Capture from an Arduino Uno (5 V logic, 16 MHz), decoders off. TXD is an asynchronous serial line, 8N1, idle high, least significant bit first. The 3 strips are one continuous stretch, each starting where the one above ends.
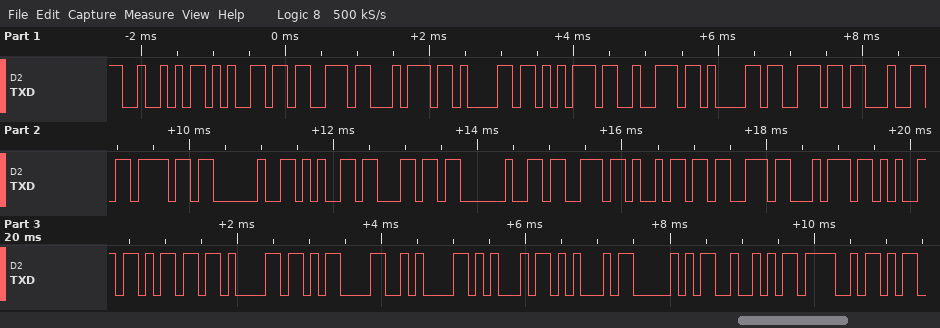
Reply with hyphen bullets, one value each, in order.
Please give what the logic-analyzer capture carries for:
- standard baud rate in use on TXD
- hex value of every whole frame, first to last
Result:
- 9600 baud
- 0x52 0x65 0x73 0x74 0x61 0x75 0x72 0x61 0x6E 0x64 0x6F 0x20 0x65 0x6C 0x20 0x73 0x69 0x73 0x74 0x65 0x6D 0x61 0x0D 0x0A 0x45 0x45 0x50 0x52 0x4F
